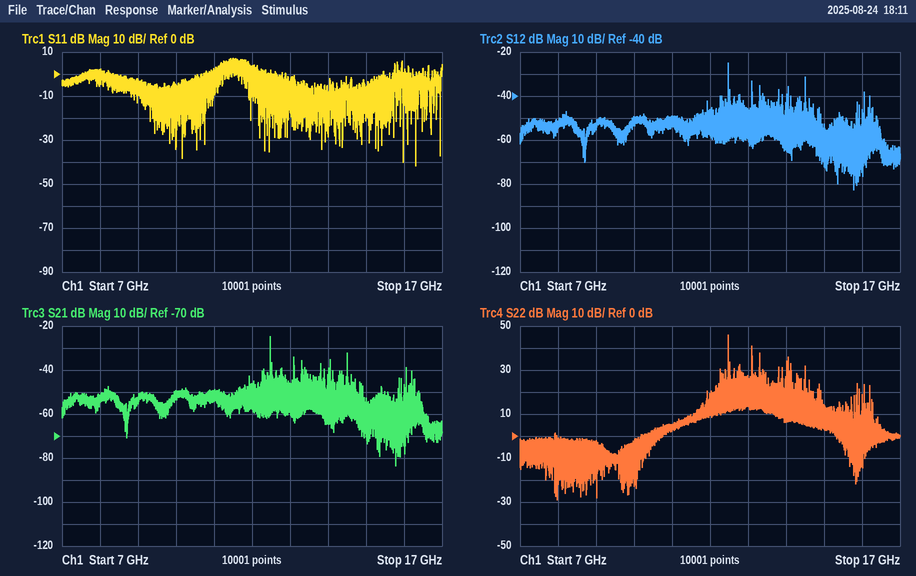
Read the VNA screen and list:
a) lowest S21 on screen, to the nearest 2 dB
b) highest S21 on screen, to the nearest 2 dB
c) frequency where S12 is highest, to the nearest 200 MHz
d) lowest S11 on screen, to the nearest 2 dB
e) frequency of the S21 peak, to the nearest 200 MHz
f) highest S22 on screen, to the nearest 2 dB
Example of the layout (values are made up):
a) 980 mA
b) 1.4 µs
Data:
a) -84 dB
b) -24 dB
c) 12.4 GHz
d) -42 dB
e) 12.4 GHz
f) 46 dB
